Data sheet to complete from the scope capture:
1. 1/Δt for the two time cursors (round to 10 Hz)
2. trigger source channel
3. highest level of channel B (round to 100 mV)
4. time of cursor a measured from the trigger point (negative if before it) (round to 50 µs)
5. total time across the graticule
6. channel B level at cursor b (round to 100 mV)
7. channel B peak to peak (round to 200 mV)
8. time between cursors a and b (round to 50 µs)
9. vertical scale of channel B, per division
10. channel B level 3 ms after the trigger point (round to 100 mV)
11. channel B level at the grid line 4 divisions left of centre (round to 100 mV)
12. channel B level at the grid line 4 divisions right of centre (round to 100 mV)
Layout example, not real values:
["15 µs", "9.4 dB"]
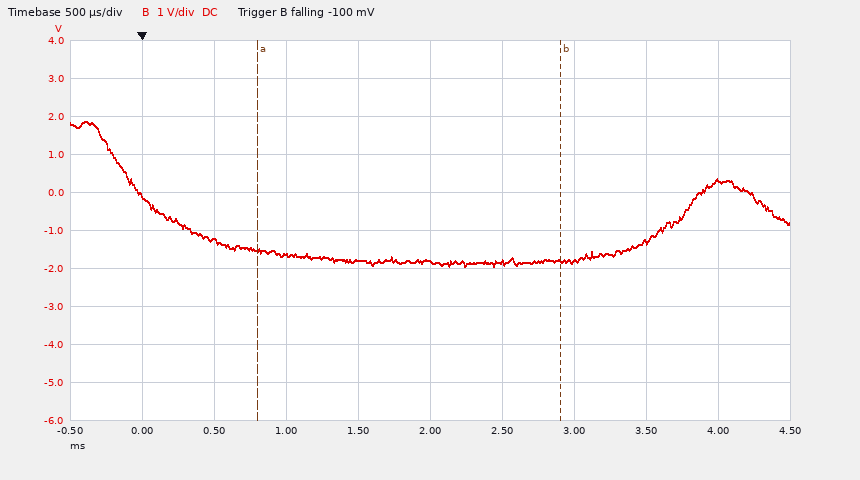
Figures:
["480 Hz", "channel B", "1.9 V", "+800 µs", "5 ms", "-1.8 V", "3.8 V", "2.10 ms", "1 V", "-1.8 V", "-100 mV", "300 mV"]
